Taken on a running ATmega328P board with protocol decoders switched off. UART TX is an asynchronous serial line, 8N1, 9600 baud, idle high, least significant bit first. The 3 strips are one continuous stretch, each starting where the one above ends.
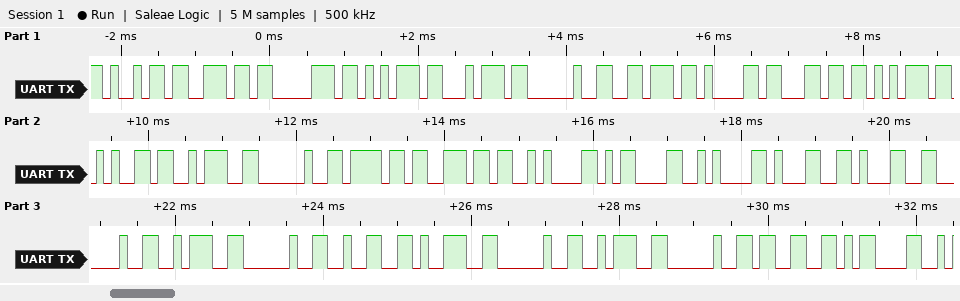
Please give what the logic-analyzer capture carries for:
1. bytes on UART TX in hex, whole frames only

69 6E 70 75 74 20 76 61 6C 75 65 3A 20 6F 6E 0A 0D 0A 31 31 20 3A 20 32 39 20 3A 20 33 0D
